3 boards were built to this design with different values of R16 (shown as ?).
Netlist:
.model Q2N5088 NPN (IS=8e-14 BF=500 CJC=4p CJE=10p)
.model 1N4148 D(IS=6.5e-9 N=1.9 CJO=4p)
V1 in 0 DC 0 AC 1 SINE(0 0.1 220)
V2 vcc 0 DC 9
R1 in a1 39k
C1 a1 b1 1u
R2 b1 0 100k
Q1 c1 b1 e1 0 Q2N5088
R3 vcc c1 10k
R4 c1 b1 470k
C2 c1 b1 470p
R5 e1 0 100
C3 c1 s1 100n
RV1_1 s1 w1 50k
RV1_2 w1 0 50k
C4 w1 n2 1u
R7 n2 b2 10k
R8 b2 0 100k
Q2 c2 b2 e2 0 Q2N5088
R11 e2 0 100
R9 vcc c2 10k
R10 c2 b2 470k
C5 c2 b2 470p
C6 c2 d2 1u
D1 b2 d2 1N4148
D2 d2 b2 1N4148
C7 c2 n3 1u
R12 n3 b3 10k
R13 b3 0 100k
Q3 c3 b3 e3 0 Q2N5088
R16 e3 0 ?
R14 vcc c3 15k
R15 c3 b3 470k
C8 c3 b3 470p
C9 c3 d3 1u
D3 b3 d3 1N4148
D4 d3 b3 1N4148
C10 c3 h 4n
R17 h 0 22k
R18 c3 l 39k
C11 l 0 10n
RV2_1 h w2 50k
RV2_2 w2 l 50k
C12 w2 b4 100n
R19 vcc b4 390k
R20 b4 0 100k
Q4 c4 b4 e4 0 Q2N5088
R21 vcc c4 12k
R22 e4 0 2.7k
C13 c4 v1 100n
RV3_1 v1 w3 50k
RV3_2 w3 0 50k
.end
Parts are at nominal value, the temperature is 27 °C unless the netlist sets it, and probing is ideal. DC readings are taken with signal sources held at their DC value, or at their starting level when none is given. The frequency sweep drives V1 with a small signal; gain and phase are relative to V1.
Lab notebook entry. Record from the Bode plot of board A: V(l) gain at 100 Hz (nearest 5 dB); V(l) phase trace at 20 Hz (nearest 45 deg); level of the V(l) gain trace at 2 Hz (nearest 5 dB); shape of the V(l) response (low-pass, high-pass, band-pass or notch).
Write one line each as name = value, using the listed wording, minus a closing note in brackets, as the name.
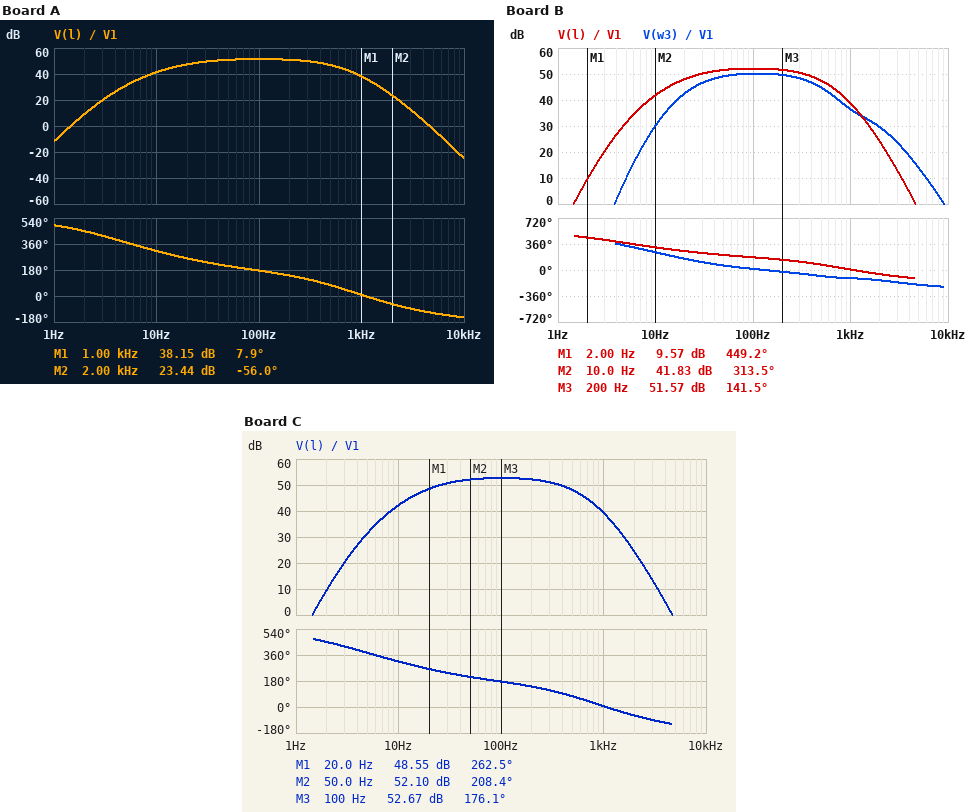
V(l) gain at 100 Hz = 50 dB
V(l) phase trace at 20 Hz = 270 deg
level of the V(l) gain trace at 2 Hz = 10 dB
shape of the V(l) response = band-pass
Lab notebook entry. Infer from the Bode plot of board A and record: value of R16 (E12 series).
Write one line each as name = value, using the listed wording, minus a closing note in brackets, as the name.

value of R16 = 270 Ω
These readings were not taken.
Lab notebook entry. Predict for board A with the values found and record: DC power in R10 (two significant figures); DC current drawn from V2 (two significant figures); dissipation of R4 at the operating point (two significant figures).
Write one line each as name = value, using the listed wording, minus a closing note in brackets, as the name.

DC power in R10 = 25 µW
DC current drawn from V2 = 1.8 mA
dissipation of R4 at the operating point = 25 µW
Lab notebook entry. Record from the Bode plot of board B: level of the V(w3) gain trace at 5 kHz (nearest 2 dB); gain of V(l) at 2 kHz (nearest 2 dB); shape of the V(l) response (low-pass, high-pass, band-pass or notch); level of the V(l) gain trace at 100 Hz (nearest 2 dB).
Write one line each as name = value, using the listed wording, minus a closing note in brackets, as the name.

level of the V(w3) gain trace at 5 kHz = 14 dB
gain of V(l) at 2 kHz = 24 dB
shape of the V(l) response = band-pass
level of the V(l) gain trace at 100 Hz = 52 dB
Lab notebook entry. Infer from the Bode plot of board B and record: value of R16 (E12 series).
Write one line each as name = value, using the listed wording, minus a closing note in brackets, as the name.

value of R16 = 220 Ω
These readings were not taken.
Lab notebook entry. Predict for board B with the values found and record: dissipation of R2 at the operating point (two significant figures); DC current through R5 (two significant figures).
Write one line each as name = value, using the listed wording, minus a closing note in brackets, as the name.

dissipation of R2 at the operating point = 4.0 µW
DC current through R5 = 490 µA
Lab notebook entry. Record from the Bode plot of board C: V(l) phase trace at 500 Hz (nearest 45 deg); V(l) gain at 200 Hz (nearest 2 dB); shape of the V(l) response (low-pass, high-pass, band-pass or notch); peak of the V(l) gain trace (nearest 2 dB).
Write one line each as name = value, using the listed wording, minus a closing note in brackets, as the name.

V(l) phase trace at 500 Hz = 90 deg
V(l) gain at 200 Hz = 52 dB
shape of the V(l) response = band-pass
peak of the V(l) gain trace = 52 dB
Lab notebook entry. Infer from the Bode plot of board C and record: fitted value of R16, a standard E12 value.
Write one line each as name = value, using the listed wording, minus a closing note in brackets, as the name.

fitted value of R16, a standard E12 value = 180 Ω
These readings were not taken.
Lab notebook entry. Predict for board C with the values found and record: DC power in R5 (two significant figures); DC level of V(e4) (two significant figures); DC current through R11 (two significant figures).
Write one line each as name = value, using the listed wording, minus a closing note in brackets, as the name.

DC power in R5 = 24 µW
DC level of V(e4) = 1.2 V
DC current through R11 = 490 µA
